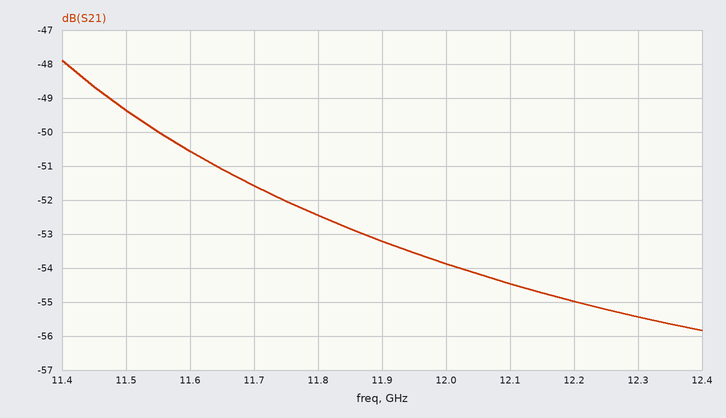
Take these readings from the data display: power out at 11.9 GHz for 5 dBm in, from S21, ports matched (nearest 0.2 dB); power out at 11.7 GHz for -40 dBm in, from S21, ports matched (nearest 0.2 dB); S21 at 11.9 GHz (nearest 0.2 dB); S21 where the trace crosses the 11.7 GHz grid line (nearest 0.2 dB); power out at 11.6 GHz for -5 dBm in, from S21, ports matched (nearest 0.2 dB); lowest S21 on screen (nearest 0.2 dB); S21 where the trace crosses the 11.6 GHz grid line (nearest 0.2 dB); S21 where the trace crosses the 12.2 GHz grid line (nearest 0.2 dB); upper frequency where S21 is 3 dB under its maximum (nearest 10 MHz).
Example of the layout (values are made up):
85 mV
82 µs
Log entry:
-48.2 dBm
-91.6 dBm
-53.2 dB
-51.6 dB
-55.6 dBm
-55.8 dB
-50.6 dB
-55.0 dB
11.63 GHz
